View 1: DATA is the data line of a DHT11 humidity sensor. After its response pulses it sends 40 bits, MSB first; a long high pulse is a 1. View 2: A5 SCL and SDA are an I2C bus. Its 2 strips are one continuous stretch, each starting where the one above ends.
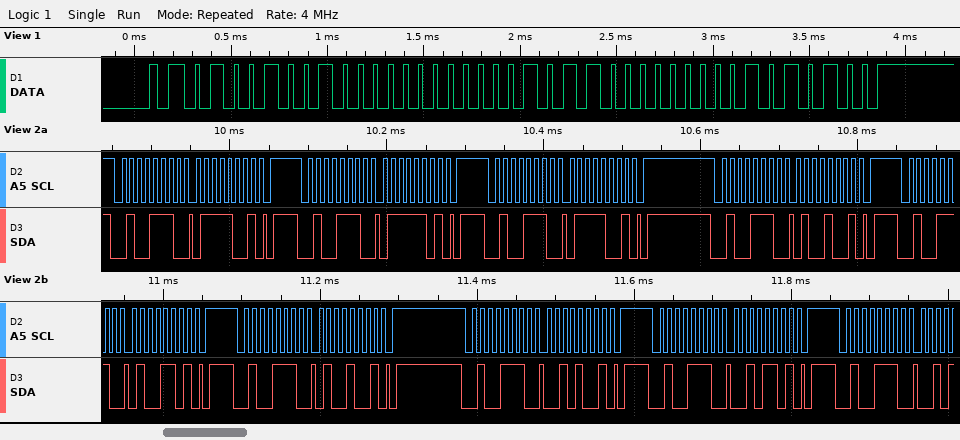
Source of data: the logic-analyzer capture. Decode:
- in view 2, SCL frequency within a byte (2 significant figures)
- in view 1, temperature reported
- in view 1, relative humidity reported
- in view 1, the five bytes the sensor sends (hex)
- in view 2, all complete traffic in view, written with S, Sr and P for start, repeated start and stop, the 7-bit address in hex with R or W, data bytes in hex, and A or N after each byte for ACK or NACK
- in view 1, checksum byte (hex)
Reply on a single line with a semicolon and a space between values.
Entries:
100 kHz; 11.0 °C; 73 %; 49 00 0B 00 54; S 27W A 79 A P S 27W A 7D A P S 27W A 79 A P S 27W A 49 A P S 27W A 4D A P S 27W A 49 A P S 27W A 29 A P S 27W A 2D A P S 27W A; 0x54
